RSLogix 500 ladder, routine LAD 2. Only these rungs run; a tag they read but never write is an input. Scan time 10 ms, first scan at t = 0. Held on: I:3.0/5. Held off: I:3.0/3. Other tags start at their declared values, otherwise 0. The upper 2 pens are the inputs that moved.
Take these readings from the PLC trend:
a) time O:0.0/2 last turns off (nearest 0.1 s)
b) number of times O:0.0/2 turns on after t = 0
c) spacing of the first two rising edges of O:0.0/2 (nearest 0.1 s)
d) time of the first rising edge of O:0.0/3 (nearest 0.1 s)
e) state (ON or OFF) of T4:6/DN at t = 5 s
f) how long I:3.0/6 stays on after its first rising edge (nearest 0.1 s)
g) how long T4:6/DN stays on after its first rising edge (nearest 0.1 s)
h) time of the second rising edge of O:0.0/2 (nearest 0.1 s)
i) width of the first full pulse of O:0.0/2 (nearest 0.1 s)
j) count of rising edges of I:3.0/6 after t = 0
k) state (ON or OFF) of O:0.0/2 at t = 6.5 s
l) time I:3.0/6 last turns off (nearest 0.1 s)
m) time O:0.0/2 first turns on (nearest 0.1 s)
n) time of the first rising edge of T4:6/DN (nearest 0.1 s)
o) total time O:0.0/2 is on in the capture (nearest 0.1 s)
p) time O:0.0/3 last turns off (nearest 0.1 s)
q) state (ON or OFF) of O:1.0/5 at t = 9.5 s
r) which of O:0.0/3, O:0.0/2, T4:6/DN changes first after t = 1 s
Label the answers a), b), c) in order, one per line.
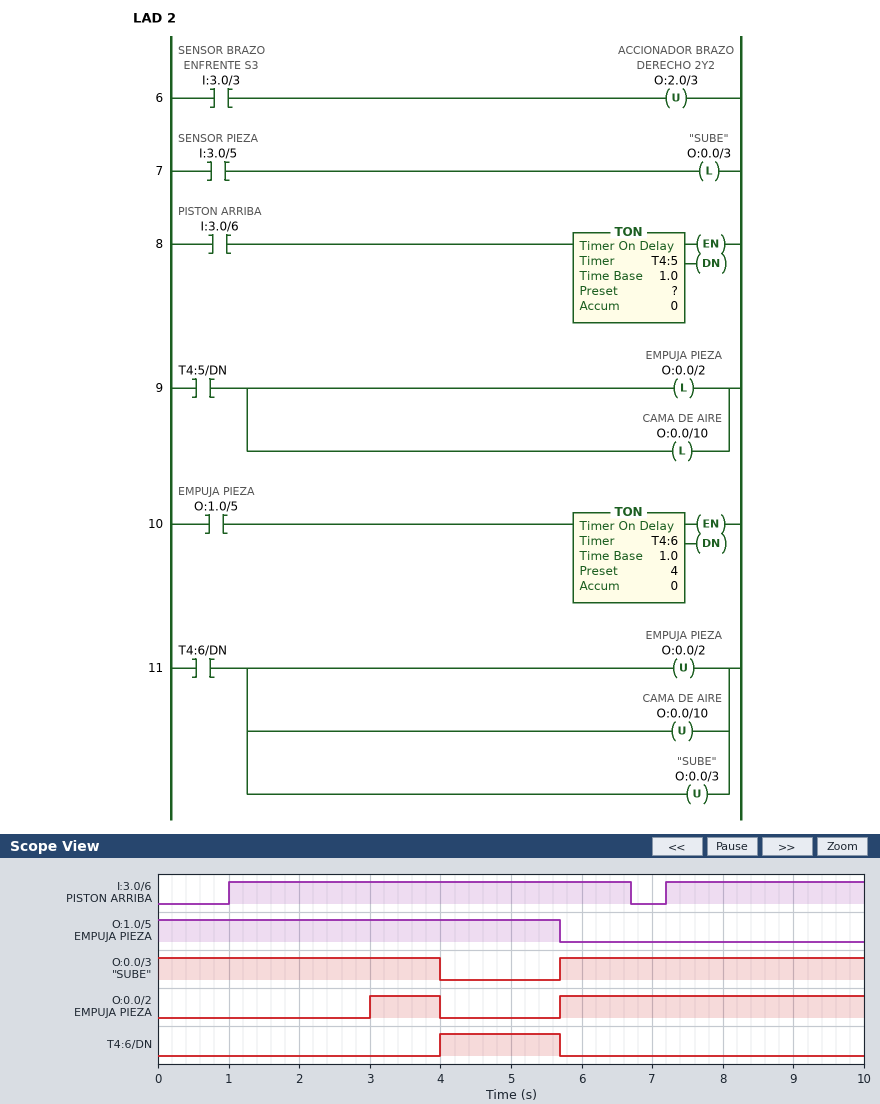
a) 4.0 s
b) 2
c) 2.7 s
d) 5.7 s
e) ON
f) 5.7 s
g) 1.7 s
h) 5.7 s
i) 1.0 s
j) 2
k) ON
l) 6.7 s
m) 3.0 s
n) 4.0 s
o) 5.3 s
p) 4.0 s
q) OFF
r) O:0.0/2
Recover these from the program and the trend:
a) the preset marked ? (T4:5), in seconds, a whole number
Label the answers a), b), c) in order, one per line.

a) 2 s
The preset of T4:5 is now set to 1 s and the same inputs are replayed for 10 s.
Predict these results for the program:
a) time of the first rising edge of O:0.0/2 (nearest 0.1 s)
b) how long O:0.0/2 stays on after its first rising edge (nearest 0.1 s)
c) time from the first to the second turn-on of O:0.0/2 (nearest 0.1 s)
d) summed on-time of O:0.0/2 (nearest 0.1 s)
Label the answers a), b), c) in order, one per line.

a) 2.0 s
b) 2.0 s
c) 3.7 s
d) 6.3 s
